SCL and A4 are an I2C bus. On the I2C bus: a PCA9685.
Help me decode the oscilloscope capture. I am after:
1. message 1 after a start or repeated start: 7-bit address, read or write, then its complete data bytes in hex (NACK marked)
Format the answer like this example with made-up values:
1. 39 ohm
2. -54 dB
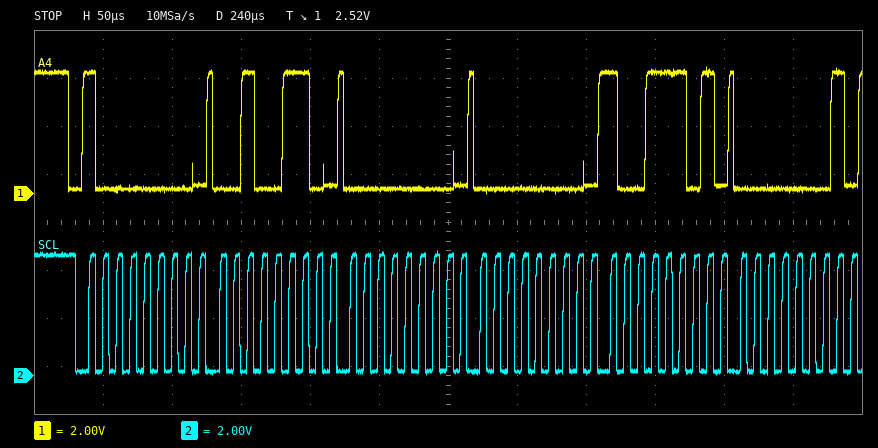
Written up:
1. 0x40 write: 26 00 00 9D 01
